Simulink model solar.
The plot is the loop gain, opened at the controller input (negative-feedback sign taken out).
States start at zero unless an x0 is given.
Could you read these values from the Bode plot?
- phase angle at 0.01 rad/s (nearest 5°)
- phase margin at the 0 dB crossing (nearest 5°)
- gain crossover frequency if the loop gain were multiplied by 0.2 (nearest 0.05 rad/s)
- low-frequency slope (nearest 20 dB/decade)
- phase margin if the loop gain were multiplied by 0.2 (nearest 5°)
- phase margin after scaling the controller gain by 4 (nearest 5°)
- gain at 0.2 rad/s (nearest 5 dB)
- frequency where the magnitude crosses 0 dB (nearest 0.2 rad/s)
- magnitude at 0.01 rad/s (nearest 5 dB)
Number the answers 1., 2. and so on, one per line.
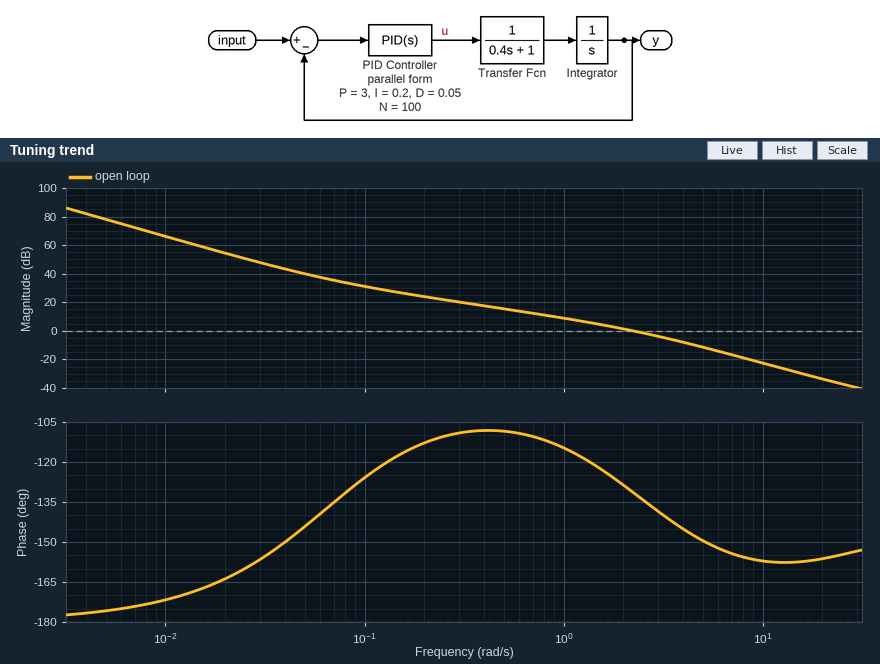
1. -170°
2. 50°
3. 0.60 rad/s
4. -40 dB/decade
5. 70°
6. 30°
7. 25 dB
8. 2.2 rad/s
9. 65 dB
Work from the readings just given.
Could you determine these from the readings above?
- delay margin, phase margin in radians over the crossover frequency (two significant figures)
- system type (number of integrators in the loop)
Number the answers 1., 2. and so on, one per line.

1. 0.40 s
2. 2
